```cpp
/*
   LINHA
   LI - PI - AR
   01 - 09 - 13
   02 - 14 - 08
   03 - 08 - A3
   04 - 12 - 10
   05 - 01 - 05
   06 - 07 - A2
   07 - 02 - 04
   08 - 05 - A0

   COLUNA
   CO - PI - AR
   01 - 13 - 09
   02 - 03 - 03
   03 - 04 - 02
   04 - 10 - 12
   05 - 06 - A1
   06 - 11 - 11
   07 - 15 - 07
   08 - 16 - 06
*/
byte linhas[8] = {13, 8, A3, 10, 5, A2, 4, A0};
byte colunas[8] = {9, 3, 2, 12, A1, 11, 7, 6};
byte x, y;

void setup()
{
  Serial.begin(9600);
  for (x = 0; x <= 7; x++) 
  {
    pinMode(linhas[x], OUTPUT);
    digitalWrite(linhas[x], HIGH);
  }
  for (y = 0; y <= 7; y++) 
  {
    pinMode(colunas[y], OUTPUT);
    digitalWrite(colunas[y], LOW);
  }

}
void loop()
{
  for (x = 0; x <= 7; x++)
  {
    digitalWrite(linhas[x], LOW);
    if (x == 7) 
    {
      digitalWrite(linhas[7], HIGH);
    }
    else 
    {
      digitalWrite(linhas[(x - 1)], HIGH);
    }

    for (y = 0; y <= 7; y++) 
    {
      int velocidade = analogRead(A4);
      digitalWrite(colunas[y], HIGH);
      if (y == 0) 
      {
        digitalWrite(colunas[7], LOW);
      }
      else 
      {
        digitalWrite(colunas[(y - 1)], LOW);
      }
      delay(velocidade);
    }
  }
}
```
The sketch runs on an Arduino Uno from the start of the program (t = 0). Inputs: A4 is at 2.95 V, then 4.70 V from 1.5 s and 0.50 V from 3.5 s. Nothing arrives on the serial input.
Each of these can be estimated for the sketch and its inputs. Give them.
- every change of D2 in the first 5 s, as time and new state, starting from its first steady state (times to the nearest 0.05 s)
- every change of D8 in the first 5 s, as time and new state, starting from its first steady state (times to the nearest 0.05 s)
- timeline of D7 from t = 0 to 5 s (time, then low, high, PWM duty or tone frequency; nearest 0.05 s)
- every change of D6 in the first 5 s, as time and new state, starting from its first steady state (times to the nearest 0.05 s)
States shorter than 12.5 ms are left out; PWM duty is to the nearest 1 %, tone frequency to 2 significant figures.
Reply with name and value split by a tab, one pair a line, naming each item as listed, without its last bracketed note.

every change of D2 in the first 5 s, as time and new state, starting from its first steady state	0 s low; 1.2 s high; 1.8 s low; 4.25 s high; 4.35 s low
every change of D8 in the first 5 s, as time and new state, starting from its first steady state	0 s high; 4.05 s low; 4.85 s high
timeline of D7 from t = 0 to 5 s	0 s low; 3.85 s high; 3.95 s low; 4.65 s high; 4.75 s low
every change of D6 in the first 5 s, as time and new state, starting from its first steady state	0 s low; 3.95 s high; 4.05 s low; 4.75 s high; 4.85 s low
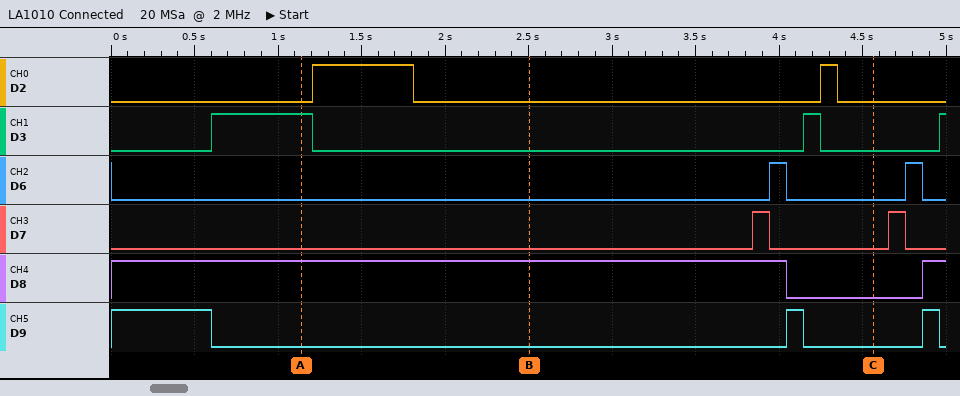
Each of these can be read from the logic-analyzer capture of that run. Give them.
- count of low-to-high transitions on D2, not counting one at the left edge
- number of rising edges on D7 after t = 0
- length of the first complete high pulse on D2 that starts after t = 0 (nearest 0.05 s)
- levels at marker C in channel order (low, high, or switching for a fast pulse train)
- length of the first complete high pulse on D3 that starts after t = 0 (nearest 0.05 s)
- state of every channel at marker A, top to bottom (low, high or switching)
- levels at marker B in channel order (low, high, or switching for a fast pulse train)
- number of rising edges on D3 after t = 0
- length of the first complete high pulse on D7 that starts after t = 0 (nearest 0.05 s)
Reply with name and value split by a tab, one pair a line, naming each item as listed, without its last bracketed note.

count of low-to-high transitions on D2, not counting one at the left edge	2
number of rising edges on D7 after t = 0	2
length of the first complete high pulse on D2 that starts after t = 0	0.60 s
levels at marker C in channel order	D2 low, D3 low, D6 low, D7 low, D8 low, D9 low
length of the first complete high pulse on D3 that starts after t = 0	0.60 s
state of every channel at marker A, top to bottom	D2 low, D3 high, D6 low, D7 low, D8 high, D9 low
levels at marker B in channel order	D2 low, D3 low, D6 low, D7 low, D8 high, D9 low
number of rising edges on D3 after t = 0	3
length of the first complete high pulse on D7 that starts after t = 0	0.10 s
